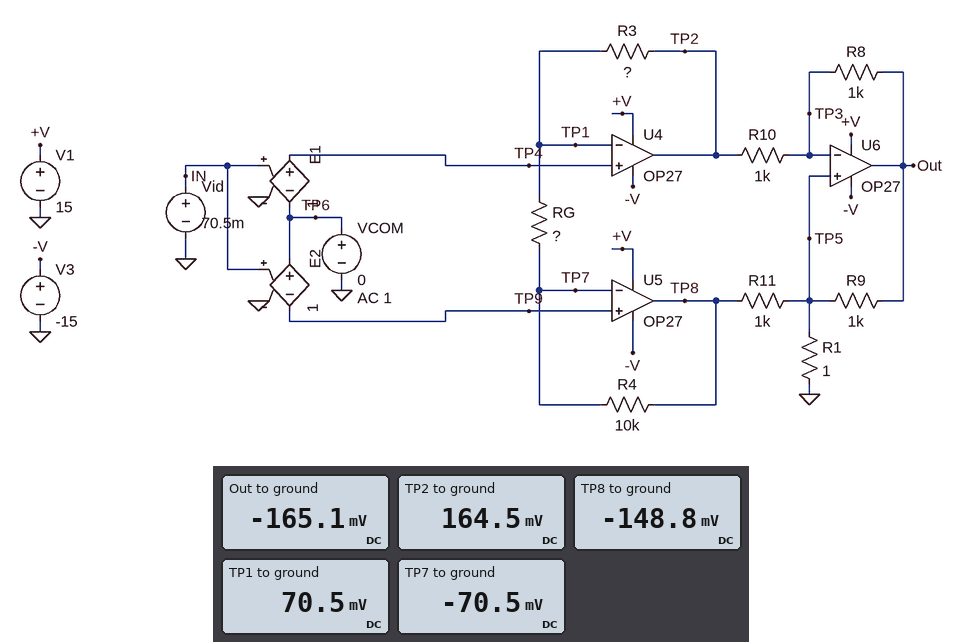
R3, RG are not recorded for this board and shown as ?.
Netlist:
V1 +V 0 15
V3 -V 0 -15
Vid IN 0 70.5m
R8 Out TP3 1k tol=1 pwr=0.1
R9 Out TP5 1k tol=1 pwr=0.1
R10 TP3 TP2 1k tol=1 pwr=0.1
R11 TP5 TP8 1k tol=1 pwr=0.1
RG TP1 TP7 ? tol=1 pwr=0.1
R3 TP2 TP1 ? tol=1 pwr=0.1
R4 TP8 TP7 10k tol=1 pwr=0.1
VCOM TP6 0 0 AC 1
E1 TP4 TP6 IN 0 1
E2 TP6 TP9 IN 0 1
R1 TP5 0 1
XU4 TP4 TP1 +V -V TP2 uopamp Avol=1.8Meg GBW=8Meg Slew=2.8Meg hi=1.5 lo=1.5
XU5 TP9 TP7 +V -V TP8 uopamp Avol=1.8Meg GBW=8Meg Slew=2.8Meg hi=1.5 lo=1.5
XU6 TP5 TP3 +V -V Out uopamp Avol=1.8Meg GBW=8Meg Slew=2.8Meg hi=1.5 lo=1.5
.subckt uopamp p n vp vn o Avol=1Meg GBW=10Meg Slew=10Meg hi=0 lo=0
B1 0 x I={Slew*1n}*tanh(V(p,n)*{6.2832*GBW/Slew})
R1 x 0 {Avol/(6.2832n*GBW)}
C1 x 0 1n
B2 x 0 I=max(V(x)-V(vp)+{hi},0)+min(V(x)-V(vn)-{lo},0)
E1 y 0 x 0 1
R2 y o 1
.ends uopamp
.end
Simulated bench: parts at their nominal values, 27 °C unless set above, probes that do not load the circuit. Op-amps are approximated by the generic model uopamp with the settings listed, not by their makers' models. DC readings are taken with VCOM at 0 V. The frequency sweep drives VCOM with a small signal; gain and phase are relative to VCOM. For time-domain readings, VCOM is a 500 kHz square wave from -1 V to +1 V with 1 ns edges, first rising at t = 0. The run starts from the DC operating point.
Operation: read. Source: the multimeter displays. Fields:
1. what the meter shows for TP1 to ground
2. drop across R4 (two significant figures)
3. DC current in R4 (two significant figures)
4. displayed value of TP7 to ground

70.5 mV
78 mV
7.8 µA
-70.5 mV
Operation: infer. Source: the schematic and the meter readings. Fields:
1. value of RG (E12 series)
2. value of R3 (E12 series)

18 kΩ
12 kΩ
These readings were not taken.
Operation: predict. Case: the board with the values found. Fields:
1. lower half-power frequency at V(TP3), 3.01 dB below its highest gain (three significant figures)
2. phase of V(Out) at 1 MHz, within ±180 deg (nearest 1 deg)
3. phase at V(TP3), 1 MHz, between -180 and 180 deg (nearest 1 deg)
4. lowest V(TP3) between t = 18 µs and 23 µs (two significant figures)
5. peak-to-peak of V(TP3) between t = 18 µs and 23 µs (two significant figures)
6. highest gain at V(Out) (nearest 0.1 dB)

2.24 MHz
159 deg
69 deg
-120 mV
230 mV
0 dB
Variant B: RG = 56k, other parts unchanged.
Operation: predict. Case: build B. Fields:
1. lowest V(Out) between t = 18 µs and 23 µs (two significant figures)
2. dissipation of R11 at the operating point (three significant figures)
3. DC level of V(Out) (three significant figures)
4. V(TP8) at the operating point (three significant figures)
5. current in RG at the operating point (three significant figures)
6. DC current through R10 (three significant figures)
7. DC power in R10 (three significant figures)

-1.1 V
9.12 µW
-101 mV
-95.7 mV
2.52 µA
101 µA
10.2 µW
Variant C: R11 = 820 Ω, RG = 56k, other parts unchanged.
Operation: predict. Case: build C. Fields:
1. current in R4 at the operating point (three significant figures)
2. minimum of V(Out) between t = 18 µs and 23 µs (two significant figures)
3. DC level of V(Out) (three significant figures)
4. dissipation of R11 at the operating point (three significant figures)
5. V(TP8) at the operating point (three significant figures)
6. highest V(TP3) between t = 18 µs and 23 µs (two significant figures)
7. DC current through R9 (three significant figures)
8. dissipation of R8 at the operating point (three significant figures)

2.52 µA
-1.1 V
-101 mV
11.1 µW
-95.7 mV
120 mV
101 µA
10.2 µW
